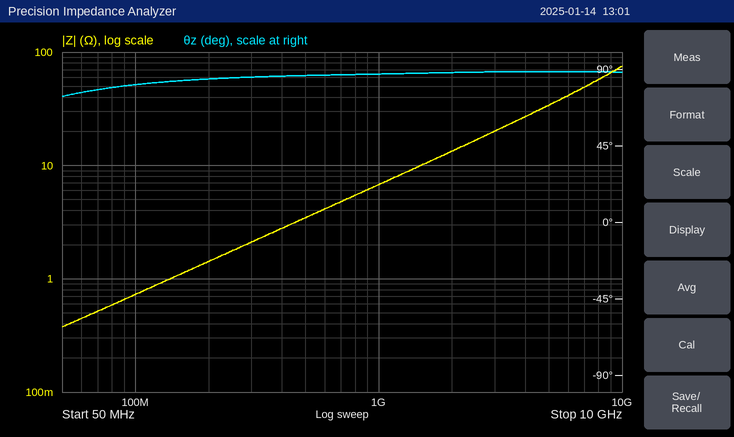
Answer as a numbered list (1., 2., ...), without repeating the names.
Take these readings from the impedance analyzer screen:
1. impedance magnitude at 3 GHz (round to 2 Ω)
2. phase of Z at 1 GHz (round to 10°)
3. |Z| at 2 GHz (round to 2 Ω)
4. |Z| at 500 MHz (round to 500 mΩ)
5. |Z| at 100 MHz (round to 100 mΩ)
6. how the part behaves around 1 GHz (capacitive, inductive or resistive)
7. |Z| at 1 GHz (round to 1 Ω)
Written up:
1. 20 Ω
2. 90°
3. 14 Ω
4. 3.5 Ω
5. 700 mΩ
6. inductive
7. 7 Ω
